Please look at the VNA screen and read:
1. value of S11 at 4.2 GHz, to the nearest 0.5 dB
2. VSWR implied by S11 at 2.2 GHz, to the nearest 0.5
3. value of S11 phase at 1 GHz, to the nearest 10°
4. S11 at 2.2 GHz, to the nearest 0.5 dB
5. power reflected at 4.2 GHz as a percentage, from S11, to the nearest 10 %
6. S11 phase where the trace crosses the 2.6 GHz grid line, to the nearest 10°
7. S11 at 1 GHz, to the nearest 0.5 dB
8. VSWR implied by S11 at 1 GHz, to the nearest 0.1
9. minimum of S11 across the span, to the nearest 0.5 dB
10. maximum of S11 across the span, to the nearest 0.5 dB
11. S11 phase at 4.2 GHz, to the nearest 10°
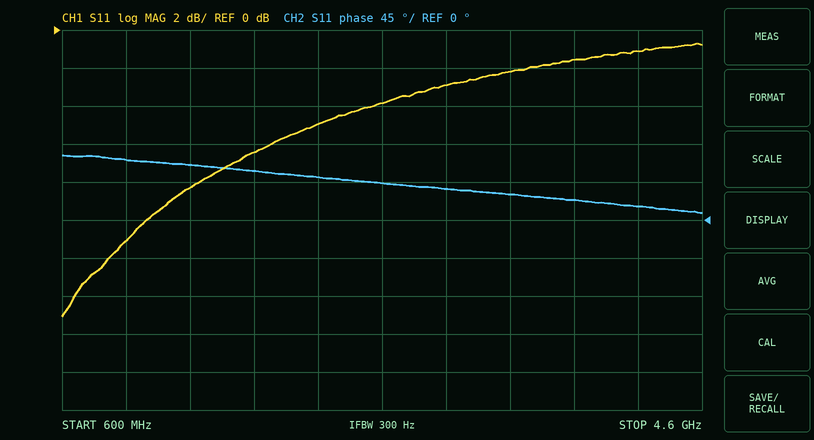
-1.0 dB
3.5
70°
-5.0 dB
80 %
40°
-11.0 dB
1.8
-15.0 dB
-0.5 dB
20°
